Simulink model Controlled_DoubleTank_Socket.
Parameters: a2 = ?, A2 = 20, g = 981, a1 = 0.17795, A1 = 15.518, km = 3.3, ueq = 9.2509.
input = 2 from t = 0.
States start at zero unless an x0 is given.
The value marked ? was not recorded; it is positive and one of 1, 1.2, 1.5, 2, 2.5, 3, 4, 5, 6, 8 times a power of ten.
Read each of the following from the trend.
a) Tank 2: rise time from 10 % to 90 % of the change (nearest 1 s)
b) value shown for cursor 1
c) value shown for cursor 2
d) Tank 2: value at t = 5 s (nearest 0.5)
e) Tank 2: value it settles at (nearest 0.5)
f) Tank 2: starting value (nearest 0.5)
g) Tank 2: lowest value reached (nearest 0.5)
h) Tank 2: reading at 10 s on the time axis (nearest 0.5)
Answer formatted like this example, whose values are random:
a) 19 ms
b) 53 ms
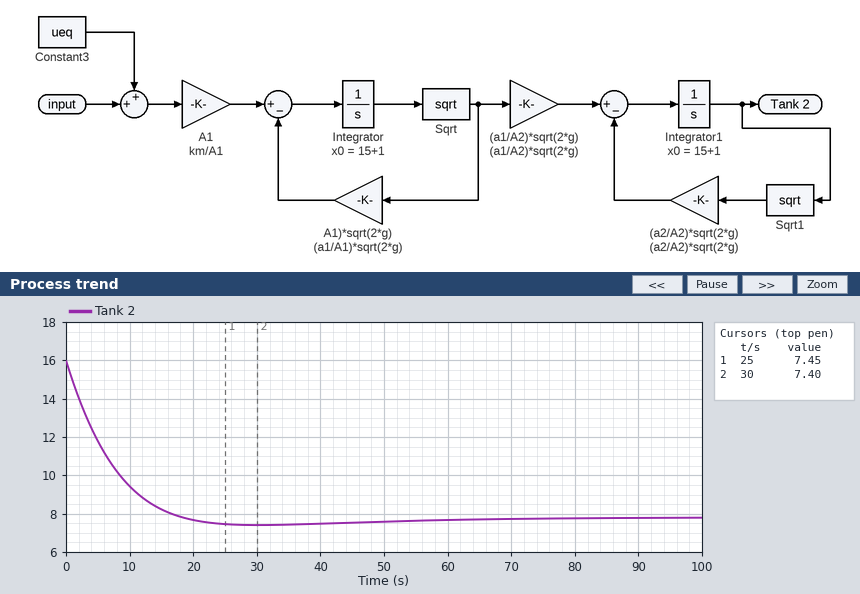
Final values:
a) 12 s
b) 7.45
c) 7.40
d) 12.0
e) 8.0
f) 16.0
g) 7.5
h) 9.5
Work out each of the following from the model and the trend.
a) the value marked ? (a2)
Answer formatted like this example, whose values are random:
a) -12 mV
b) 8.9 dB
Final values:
a) 0.3
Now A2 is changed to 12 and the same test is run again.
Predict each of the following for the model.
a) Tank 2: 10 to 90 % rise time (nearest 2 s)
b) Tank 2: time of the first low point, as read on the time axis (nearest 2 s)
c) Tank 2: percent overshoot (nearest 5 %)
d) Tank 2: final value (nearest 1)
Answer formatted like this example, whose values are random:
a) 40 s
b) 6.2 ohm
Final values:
a) 6 s
b) 18 s
c) 10 %
d) 8
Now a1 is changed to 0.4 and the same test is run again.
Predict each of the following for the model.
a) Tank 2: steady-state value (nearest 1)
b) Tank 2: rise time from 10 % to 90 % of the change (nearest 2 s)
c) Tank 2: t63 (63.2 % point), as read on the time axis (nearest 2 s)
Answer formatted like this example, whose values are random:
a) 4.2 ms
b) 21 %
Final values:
a) 8
b) 22 s
c) 20 s
